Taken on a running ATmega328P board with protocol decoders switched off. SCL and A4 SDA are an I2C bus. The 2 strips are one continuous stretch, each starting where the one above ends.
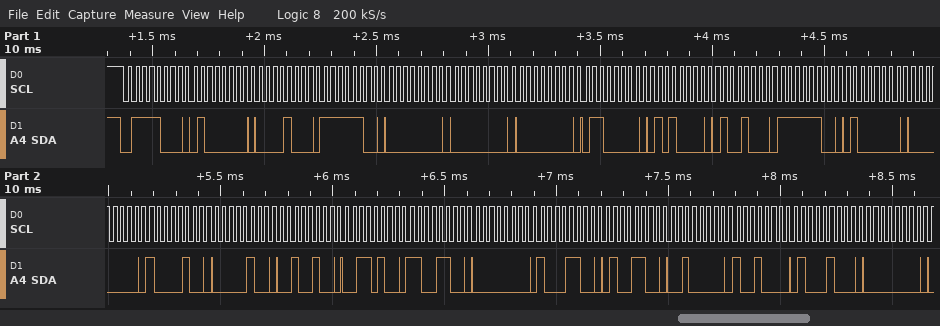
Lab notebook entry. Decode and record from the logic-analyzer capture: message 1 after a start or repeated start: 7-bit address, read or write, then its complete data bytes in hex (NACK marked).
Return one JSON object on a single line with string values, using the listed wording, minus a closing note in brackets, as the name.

{"message 1 after a start or repeated start: 7-bit address, read or write, then its complete data bytes in hex": "0x3C write: 40 08 FC 00 00 00 60 50 48 FC 40 00 84 04 24 34 CC 00 8C 4C 20 90 88 00"}
